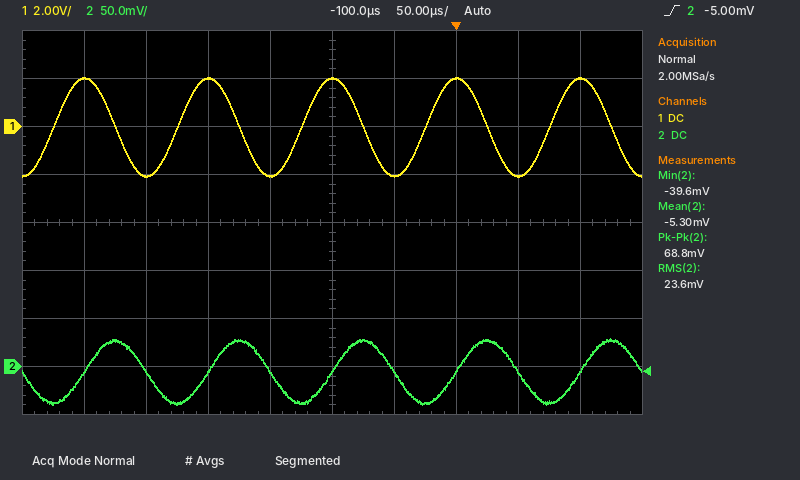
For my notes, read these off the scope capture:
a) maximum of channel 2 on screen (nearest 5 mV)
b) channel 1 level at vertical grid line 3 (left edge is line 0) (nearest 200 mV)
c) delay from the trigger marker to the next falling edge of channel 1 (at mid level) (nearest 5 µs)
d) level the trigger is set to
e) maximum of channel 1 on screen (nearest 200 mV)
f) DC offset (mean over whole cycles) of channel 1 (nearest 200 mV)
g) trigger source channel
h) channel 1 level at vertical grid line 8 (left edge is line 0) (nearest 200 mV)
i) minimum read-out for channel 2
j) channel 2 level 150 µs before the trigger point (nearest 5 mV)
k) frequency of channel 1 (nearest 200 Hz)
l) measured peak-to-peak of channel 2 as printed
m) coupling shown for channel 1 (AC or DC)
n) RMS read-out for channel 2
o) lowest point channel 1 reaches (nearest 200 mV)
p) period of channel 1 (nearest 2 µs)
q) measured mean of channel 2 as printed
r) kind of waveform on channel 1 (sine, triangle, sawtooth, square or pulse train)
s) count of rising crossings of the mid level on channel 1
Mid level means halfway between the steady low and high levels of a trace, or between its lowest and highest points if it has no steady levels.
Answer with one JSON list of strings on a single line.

["30 mV", "2.0 V", "25 µs", "-5.00 mV", "2.0 V", "0.0 V", "channel 2", "-2.0 V", "-39.6 mV", "-5 mV", "10.0 kHz", "68.8 mV", "DC", "23.6 mV", "-2.0 V", "100 µs", "-5.30 mV", "sine", "5"]
